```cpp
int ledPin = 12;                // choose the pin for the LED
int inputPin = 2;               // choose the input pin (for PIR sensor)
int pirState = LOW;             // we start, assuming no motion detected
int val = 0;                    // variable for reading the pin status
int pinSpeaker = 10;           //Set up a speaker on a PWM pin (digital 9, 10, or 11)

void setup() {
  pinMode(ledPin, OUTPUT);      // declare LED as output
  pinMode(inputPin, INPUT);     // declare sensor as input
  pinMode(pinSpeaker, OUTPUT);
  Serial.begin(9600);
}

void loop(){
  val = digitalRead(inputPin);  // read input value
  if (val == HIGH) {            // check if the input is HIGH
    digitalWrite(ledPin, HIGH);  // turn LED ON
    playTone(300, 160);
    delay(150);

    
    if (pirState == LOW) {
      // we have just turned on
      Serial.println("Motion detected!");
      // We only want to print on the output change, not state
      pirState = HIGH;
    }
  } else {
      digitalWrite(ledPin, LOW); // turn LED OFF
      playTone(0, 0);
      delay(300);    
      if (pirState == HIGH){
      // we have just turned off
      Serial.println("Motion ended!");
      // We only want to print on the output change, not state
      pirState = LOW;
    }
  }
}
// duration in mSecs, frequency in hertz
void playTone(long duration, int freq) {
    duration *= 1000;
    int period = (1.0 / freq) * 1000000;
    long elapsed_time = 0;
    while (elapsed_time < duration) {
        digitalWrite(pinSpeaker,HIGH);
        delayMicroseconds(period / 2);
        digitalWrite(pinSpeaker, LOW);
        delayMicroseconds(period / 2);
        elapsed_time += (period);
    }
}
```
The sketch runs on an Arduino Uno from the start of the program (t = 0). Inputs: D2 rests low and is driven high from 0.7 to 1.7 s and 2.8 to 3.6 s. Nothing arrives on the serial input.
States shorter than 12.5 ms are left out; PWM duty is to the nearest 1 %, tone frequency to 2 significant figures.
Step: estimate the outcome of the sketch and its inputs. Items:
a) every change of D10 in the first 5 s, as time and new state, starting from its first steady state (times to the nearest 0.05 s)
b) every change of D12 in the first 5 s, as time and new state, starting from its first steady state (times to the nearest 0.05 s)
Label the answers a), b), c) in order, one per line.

a) 0 s low; 0.9 s tone 160 Hz; 1.2 s low; 1.35 s tone 160 Hz; 1.65 s low; 3 s tone 160 Hz; 3.3 s low; 3.45 s tone 160 Hz; 3.75 s low
b) 0 s low; 0.9 s high; 1.8 s low; 3 s high; 3.9 s low
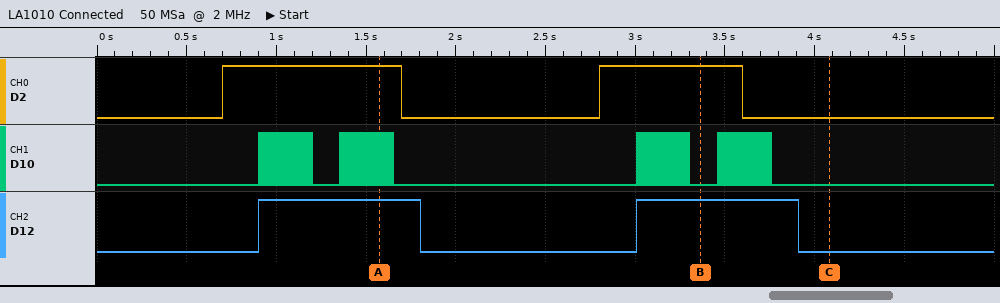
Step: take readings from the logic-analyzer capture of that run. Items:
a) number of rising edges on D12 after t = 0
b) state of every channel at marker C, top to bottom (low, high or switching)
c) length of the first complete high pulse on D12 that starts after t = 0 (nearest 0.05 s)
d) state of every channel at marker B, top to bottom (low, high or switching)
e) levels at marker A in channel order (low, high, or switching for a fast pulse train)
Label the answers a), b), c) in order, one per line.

a) 2
b) D2 low, D10 low, D12 low
c) 0.90 s
d) D2 high, D10 low, D12 high
e) D2 high, D10 switching, D12 high
